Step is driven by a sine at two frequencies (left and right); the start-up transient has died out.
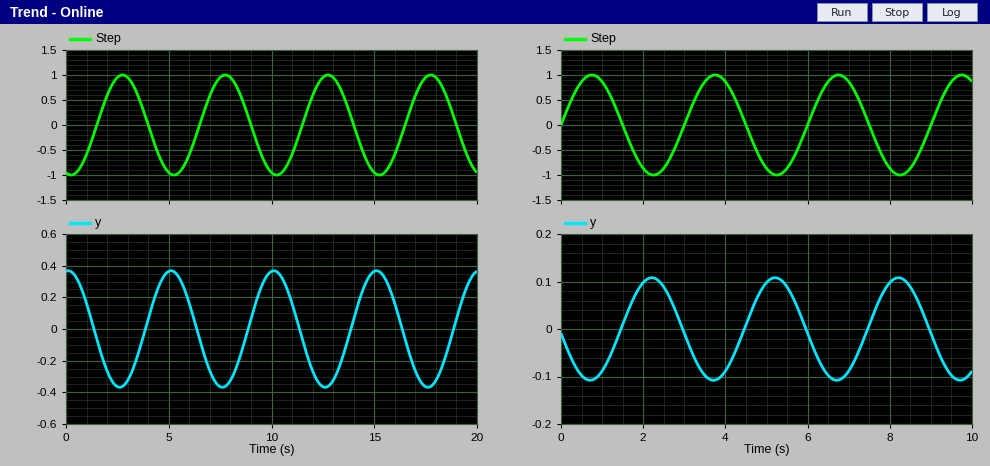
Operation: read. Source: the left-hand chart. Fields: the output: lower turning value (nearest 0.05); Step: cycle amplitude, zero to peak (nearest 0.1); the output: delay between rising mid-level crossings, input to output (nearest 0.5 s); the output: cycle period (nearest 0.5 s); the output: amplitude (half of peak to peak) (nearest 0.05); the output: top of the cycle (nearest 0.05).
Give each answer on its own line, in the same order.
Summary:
-0.35
1.0
2.5 s
5.0 s
0.35
0.35
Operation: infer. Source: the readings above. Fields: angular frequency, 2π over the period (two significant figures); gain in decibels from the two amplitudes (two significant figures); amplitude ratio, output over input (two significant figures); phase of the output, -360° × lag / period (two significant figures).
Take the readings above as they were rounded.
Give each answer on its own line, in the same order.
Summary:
1.3 rad/s
-9.1 dB
0.35
-180°
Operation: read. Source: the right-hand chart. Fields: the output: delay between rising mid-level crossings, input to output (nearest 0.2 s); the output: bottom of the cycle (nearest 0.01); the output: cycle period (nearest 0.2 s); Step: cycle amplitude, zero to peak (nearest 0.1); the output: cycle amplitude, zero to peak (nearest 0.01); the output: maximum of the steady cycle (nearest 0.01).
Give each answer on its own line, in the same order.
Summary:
1.4 s
-0.11
3.0 s
1.0
0.11
0.11
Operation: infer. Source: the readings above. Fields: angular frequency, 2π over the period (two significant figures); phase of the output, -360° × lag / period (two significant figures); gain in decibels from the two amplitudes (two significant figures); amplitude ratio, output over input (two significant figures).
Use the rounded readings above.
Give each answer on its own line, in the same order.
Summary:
2.1 rad/s
-170°
-19 dB
0.11
